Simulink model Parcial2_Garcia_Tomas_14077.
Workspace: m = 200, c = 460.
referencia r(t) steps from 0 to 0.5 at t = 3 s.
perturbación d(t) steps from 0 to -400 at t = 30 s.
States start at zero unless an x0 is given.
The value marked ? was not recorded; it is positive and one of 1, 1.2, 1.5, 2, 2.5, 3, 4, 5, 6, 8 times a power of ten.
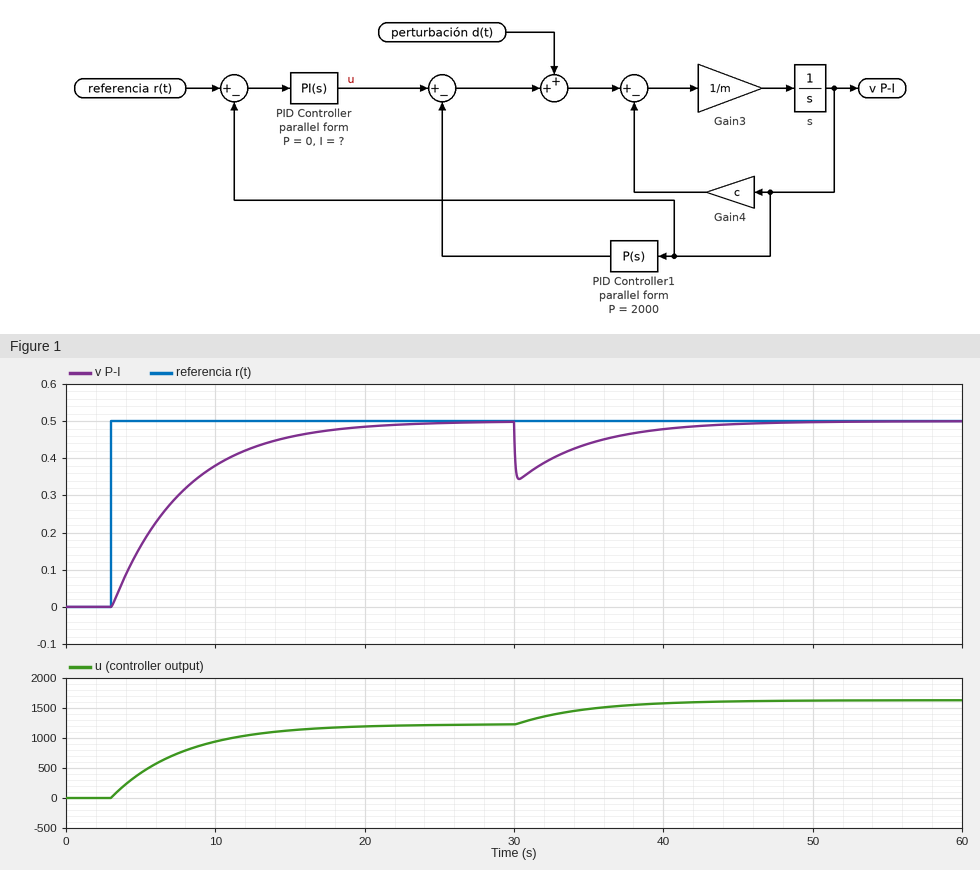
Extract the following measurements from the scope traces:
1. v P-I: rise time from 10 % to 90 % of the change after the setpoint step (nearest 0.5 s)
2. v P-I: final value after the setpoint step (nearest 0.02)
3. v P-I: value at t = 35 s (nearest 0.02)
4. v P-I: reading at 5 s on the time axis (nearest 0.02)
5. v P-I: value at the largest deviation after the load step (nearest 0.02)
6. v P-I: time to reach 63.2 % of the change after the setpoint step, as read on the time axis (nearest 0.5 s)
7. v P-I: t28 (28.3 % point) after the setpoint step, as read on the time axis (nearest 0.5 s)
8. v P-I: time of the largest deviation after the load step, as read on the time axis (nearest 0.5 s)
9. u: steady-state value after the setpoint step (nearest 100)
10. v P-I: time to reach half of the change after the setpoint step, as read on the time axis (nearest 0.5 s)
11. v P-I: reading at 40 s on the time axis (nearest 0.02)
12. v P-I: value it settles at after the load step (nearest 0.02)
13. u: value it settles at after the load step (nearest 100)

10.5 s
0.50
0.44
0.16
0.34
8.0 s
4.5 s
30.5 s
1200
6.5 s
0.48
0.50
1600
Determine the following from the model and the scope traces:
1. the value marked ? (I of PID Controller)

500
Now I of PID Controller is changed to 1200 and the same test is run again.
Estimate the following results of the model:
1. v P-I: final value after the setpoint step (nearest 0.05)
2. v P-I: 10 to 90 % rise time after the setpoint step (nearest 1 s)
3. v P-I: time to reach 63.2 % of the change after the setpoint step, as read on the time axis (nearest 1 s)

0.50
4 s
5 s
